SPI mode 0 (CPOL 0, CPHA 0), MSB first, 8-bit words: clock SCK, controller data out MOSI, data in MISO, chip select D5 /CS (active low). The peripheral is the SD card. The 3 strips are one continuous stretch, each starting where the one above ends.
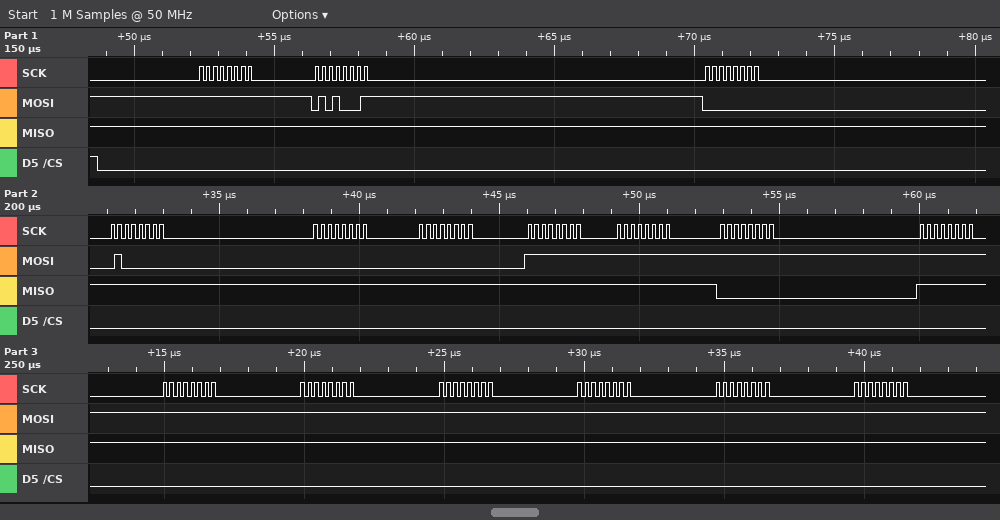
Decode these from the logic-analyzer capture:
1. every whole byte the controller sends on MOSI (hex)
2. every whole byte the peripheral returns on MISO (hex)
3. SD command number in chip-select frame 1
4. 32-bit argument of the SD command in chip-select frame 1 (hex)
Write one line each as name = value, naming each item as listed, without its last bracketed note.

every whole byte the controller sends on MOSI = 0xFF 0x51 0x00 0x40 0x00 0x00 0xFF 0xFF 0xFF 0xFF 0xFF 0xFF 0xFF 0xFF 0xFF 0xFF
every whole byte the peripheral returns on MISO = 0xFF 0xFF 0xFF 0xFF 0xFF 0xFF 0xFF 0xFF 0x00 0xFF 0xFF 0xFF 0xFF 0xFF 0xFF 0xFF
SD command number in chip-select frame 1 = CMD17
32-bit argument of the SD command in chip-select frame 1 = 0x00400000
